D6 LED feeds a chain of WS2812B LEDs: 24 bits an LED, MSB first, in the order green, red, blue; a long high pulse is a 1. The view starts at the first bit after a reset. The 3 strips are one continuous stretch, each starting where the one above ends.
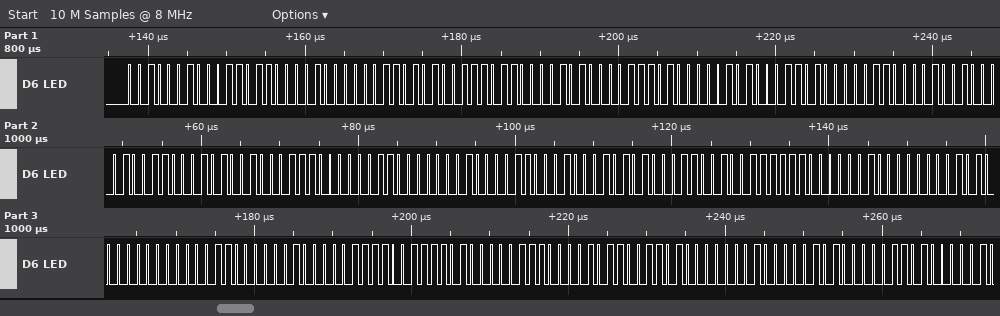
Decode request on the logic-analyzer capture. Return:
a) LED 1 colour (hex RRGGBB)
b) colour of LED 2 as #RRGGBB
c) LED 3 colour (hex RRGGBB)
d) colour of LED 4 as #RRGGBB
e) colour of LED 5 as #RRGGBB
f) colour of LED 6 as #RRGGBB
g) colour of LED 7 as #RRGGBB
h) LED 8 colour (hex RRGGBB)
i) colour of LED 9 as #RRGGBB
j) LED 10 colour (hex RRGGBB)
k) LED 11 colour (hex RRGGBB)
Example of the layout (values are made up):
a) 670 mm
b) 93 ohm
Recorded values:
a) #362210
b) #3B350A
c) #051D1A
d) #240C26
e) #1C290C
f) #310415
g) #3F1902
h) #400103
i) #0F023D
j) #0B0734
k) #14041A
